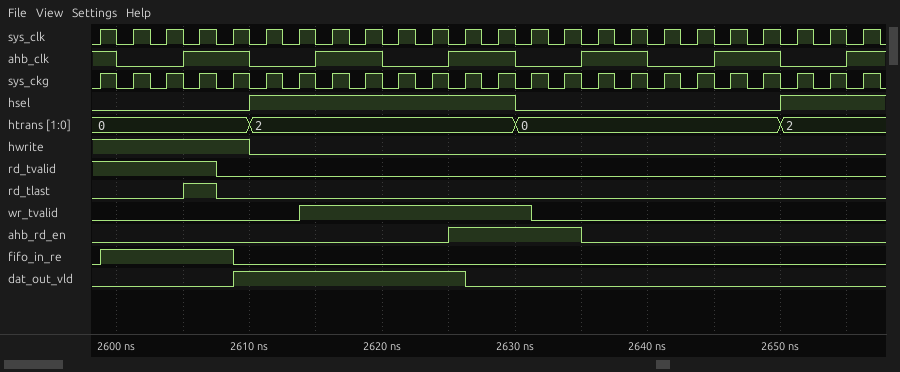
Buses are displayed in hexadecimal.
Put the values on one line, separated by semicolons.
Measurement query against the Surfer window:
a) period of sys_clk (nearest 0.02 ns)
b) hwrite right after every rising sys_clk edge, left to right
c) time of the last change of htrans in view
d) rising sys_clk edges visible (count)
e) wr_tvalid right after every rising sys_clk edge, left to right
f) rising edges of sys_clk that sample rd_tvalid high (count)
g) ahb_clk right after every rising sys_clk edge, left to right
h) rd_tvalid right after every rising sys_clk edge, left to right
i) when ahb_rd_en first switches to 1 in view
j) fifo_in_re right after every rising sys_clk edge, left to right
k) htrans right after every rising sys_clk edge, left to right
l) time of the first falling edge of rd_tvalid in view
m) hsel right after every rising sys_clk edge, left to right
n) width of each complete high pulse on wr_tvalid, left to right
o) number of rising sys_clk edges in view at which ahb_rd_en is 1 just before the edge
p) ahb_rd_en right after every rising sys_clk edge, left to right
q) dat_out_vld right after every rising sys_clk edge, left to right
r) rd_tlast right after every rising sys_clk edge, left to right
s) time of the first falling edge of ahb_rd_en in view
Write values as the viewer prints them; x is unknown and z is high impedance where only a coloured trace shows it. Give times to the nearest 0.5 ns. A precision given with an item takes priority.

2.5 ns; 1 1 1 1 1 0 0 0 0 0 0 0 0 0 0 0 0 0 0 0 0 0 0 0; 2650 ns; 24; 0 0 0 0 0 0 1 1 1 1 1 1 1 0 0 0 0 0 0 0 0 0 0 0; 4; 1 0 0 1 1 0 0 1 1 0 0 1 1 0 0 1 1 0 0 1 1 0 0 1; 1 1 1 1 0 0 0 0 0 0 0 0 0 0 0 0 0 0 0 0 0 0 0 0; 2625 ns; 1 1 1 1 0 0 0 0 0 0 0 0 0 0 0 0 0 0 0 0 0 0 0 0; 0, 0, 0, 0, 0, 2, 2, 2, 2, 2, 2, 2, 2, 0, 0, 0, 0, 0, 0, 0, 0, 2, 2, 2; 2607.5 ns; 0 0 0 0 0 1 1 1 1 1 1 1 1 0 0 0 0 0 0 0 0 1 1 1; 17.5 ns; 4; 0 0 0 0 0 0 0 0 0 0 0 1 1 1 1 0 0 0 0 0 0 0 0 0; 0 0 0 0 1 1 1 1 1 1 1 0 0 0 0 0 0 0 0 0 0 0 0 0; 0 0 0 1 0 0 0 0 0 0 0 0 0 0 0 0 0 0 0 0 0 0 0 0; 2635 ns
